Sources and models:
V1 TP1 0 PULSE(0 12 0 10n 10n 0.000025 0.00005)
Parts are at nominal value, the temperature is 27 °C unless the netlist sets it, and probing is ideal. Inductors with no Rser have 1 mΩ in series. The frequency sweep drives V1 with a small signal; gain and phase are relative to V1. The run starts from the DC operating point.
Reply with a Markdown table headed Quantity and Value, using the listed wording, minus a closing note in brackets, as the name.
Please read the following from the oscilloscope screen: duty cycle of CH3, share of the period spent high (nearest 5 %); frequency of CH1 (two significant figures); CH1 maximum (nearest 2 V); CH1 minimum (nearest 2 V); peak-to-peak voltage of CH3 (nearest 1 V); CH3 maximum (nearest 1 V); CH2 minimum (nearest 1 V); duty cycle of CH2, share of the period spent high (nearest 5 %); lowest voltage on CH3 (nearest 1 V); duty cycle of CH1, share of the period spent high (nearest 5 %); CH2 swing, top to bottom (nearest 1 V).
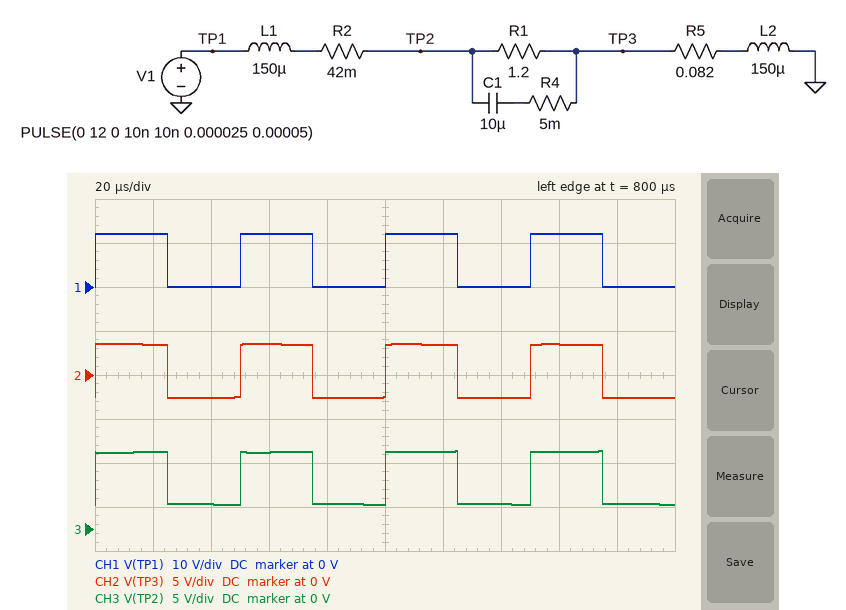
| Quantity | Value |
|---|---|
| duty cycle of CH3, share of the period spent high | 50 % |
| frequency of CH1 | 20 kHz |
| CH1 maximum | 12 V |
| CH1 minimum | 0 V |
| peak-to-peak voltage of CH3 | 6 V |
| CH3 maximum | 9 V |
| CH2 minimum | -3 V |
| duty cycle of CH2, share of the period spent high | 50 % |
| lowest voltage on CH3 | 3 V |
| duty cycle of CH1, share of the period spent high | 50 % |
| CH2 swing, top to bottom | 6 V |
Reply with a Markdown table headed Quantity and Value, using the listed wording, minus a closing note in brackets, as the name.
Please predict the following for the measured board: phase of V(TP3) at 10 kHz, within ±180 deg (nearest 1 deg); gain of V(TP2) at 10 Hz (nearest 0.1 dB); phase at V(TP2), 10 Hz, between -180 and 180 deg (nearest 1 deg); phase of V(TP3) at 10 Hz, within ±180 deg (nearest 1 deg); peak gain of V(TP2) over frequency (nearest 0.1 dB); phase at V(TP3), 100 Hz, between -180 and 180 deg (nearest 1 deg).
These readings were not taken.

| Quantity | Value |
|---|---|
| phase of V(TP3) at 10 kHz, within ±180 deg | 2 deg |
| gain of V(TP2) at 10 Hz | -0.3 dB |
| phase at V(TP2), 10 Hz, between -180 and 180 deg | 0 deg |
| phase of V(TP3) at 10 Hz, within ±180 deg | 6 deg |
| peak gain of V(TP2) over frequency | -0.3 dB |
| phase at V(TP3), 100 Hz, between -180 and 180 deg | 41 deg |
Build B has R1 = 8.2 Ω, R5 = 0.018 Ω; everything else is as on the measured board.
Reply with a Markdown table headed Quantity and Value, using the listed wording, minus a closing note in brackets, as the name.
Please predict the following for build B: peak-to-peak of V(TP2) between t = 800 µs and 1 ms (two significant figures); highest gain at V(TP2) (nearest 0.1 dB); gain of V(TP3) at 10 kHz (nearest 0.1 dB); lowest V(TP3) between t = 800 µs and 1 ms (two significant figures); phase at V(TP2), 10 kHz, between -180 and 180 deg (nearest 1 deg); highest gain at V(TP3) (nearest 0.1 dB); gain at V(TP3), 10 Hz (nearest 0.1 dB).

| Quantity | Value |
|---|---|
| peak-to-peak of V(TP2) between t = 800 µs and 1 ms | 6.0 V |
| highest gain at V(TP2) | 1.1 dB |
| gain of V(TP3) at 10 kHz | -5.3 dB |
| lowest V(TP3) between t = 800 µs and 1 ms | -3.1 V |
| phase at V(TP2), 10 kHz, between -180 and 180 deg | -1 deg |
| highest gain at V(TP3) | -0.8 dB |
| gain at V(TP3), 10 Hz | -51.8 dB |
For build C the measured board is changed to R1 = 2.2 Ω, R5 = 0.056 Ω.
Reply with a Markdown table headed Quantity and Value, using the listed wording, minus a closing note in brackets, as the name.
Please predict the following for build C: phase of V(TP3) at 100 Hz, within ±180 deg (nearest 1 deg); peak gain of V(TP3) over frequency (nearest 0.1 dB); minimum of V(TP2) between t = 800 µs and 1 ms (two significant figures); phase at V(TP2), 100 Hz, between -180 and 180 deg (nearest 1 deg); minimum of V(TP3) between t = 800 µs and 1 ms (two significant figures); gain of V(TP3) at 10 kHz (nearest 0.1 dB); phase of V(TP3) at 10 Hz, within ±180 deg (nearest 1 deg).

| Quantity | Value |
|---|---|
| phase of V(TP3) at 100 Hz, within ±180 deg | 55 deg |
| peak gain of V(TP3) over frequency | -5.2 dB |
| minimum of V(TP2) between t = 800 µs and 1 ms | 2.9 V |
| phase at V(TP2), 100 Hz, between -180 and 180 deg | -2 deg |
| minimum of V(TP3) between t = 800 µs and 1 ms | -2.9 V |
| gain of V(TP3) at 10 kHz | -5.5 dB |
| phase of V(TP3) at 10 Hz, within ±180 deg | 9 deg |
